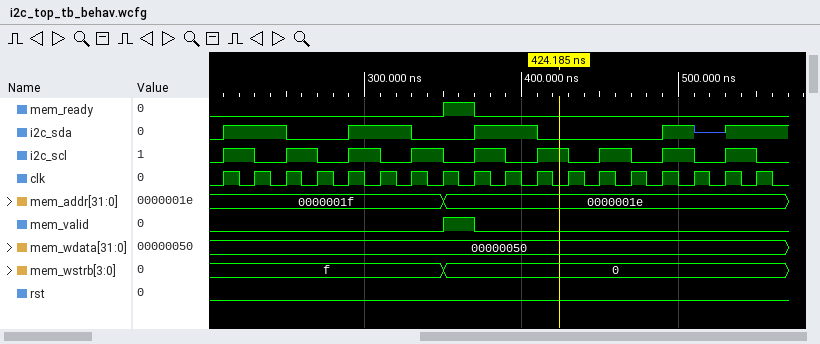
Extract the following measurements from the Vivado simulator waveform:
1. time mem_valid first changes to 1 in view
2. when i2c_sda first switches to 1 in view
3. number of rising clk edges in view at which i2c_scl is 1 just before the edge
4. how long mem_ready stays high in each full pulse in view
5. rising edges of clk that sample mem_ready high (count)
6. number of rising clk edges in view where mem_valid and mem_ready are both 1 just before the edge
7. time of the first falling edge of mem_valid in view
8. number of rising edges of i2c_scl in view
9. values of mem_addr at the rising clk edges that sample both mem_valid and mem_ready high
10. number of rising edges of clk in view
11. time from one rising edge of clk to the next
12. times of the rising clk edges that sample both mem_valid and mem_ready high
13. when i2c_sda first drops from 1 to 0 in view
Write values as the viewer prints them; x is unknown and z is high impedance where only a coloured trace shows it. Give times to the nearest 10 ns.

350 ns
210 ns
9
20 ns
1
1
370 ns
9
0000001e
18
20 ns
370 ns
250 ns
